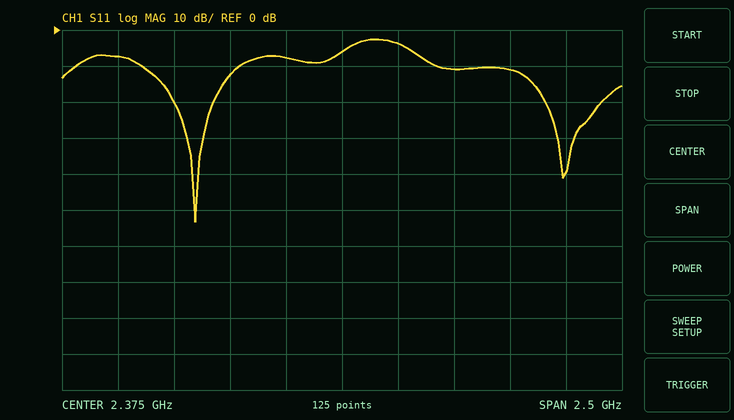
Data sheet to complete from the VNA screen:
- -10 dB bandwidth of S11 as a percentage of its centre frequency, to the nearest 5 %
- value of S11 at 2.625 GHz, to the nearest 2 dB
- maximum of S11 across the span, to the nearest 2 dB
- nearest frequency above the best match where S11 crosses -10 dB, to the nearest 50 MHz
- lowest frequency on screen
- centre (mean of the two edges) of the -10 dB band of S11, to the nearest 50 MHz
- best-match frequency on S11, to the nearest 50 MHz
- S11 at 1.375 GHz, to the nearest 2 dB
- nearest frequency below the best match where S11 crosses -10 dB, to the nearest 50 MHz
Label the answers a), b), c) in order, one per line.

a) 25 %
b) -4 dB
c) -2 dB
d) 1.90 GHz
e) 1.125 GHz
f) 1.70 GHz
g) 1.70 GHz
h) -8 dB
i) 1.50 GHz
